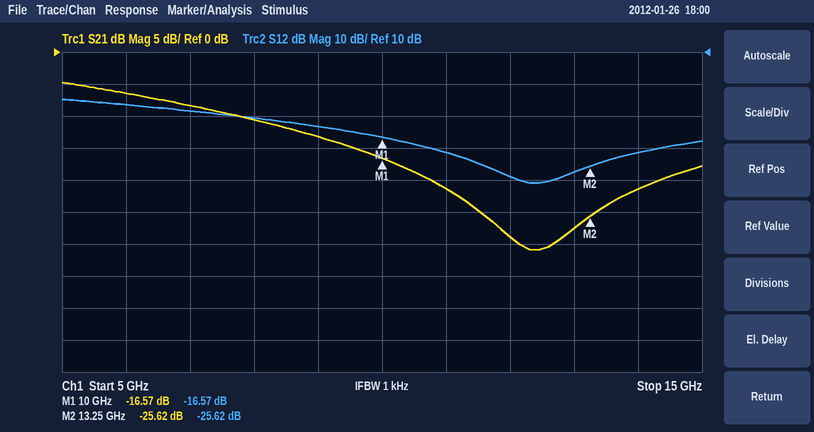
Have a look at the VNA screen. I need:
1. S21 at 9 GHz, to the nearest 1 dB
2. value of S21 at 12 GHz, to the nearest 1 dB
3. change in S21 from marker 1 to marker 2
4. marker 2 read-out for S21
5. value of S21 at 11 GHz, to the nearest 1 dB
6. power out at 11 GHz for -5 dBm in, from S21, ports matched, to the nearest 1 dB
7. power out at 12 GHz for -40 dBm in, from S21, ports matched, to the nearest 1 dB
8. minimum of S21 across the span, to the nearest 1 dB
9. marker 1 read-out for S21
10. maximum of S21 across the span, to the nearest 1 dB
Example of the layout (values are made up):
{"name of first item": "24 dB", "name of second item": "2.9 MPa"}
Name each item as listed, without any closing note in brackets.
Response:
{"S21 at 9 GHz, to the nearest 1 dB": "-13 dB", "value of S21 at 12 GHz, to the nearest 1 dB": "-29 dB", "change in S21 from marker 1 to marker 2": "-9.05 dB", "marker 2 read-out for S21": "-25.62 dB", "value of S21 at 11 GHz, to the nearest 1 dB": "-21 dB", "power out at 11 GHz for -5 dBm in, from S21, ports matched, to the nearest 1 dB": "-26 dBm", "power out at 12 GHz for -40 dBm in, from S21, ports matched, to the nearest 1 dB": "-69 dBm", "minimum of S21 across the span, to the nearest 1 dB": "-31 dB", "marker 1 read-out for S21": "-16.57 dB", "maximum of S21 across the span, to the nearest 1 dB": "-5 dB"}
